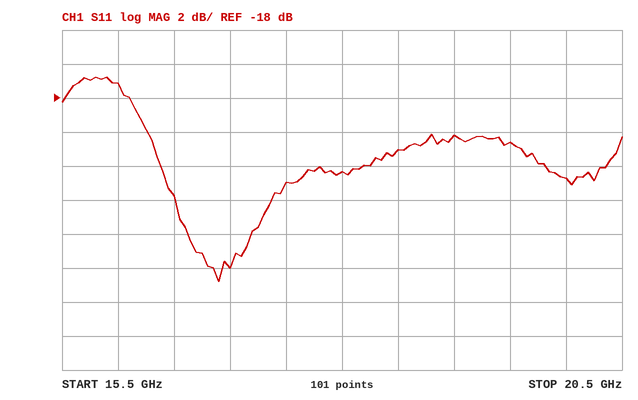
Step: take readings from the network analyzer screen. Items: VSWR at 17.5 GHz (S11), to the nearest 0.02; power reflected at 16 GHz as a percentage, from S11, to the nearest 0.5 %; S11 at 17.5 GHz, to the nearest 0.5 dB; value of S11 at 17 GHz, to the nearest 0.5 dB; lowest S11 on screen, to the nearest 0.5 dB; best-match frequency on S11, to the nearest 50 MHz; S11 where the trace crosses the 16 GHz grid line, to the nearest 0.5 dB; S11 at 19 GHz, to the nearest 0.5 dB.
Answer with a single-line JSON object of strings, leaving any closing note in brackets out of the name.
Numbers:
{"VSWR at 17.5 GHz (S11), to the nearest 0.02": "1.16", "power reflected at 16 GHz as a percentage, from S11, to the nearest 0.5 %": "2.0 %", "S11 at 17.5 GHz, to the nearest 0.5 dB": "-23.0 dB", "value of S11 at 17 GHz, to the nearest 0.5 dB": "-28.0 dB", "lowest S11 on screen, to the nearest 0.5 dB": "-29.0 dB", "best-match frequency on S11, to the nearest 50 MHz": "16.90 GHz", "S11 where the trace crosses the 16 GHz grid line, to the nearest 0.5 dB": "-17.0 dB", "S11 at 19 GHz, to the nearest 0.5 dB": "-20.0 dB"}
